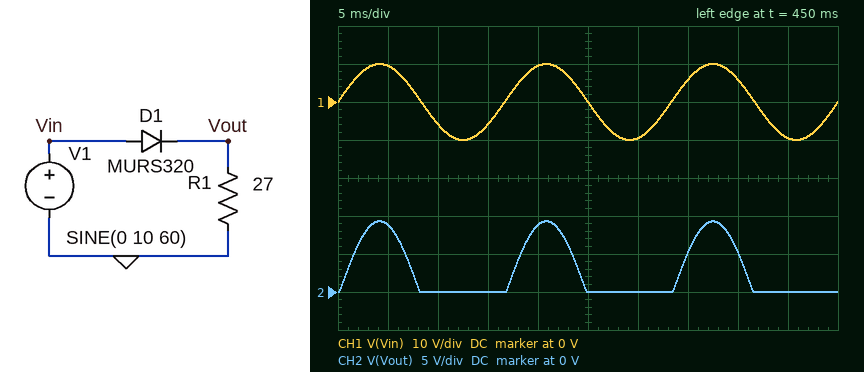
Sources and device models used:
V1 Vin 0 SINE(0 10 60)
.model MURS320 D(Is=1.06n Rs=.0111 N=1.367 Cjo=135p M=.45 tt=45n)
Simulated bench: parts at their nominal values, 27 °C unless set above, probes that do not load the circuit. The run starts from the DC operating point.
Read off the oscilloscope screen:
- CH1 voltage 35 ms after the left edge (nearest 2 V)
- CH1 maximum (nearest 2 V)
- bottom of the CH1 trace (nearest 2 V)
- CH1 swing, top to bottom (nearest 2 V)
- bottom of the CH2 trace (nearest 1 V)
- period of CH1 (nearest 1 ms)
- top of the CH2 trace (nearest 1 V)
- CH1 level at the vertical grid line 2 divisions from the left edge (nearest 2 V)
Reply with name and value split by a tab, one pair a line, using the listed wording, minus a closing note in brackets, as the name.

CH1 voltage 35 ms after the left edge	6 V
CH1 maximum	10 V
bottom of the CH1 trace	-10 V
CH1 swing, top to bottom	20 V
bottom of the CH2 trace	0 V
period of CH1	17 ms
top of the CH2 trace	9 V
CH1 level at the vertical grid line 2 divisions from the left edge	-6 V
